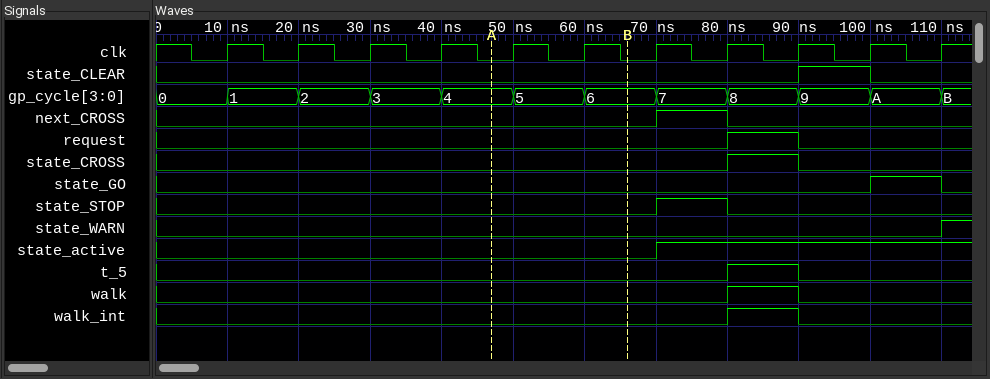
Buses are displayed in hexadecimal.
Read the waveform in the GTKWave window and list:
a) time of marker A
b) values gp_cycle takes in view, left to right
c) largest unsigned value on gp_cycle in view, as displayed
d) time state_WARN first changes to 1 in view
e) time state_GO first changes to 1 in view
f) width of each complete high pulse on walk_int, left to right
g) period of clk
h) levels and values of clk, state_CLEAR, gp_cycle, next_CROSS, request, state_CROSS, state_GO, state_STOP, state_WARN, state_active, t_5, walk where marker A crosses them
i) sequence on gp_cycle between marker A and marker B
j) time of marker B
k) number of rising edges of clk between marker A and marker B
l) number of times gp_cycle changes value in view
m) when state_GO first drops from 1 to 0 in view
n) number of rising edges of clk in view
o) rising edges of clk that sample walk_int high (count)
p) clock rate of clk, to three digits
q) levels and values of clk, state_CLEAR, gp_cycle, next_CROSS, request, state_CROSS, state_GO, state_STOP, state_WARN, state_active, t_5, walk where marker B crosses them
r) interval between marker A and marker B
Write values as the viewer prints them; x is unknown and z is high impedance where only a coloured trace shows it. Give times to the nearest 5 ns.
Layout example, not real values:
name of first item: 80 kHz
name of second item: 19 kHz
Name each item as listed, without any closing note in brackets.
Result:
time of marker A: 45 ns
values gp_cycle takes in view, left to right: 0, 1, 2, 3, 4, 5, 6, 7, 8, 9, A, B
largest unsigned value on gp_cycle in view, as displayed: B
time state_WARN first changes to 1 in view: 110 ns
time state_GO first changes to 1 in view: 100 ns
width of each complete high pulse on walk_int, left to right: 10 ns
period of clk: 10 ns
levels and values of clk, state_CLEAR, gp_cycle, next_CROSS, request, state_CROSS, state_GO, state_STOP, state_WARN, state_active, t_5, walk where marker A crosses them: clk=0, state_CLEAR=0, gp_cycle=4, next_CROSS=0, request=0, state_CROSS=0, state_GO=0, state_STOP=0, state_WARN=0, state_active=0, t_5=0, walk=0
sequence on gp_cycle between marker A and marker B: 4, 5, 6
time of marker B: 65 ns
number of rising edges of clk between marker A and marker B: 2
number of times gp_cycle changes value in view: 11
when state_GO first drops from 1 to 0 in view: 110 ns
number of rising edges of clk in view: 11
rising edges of clk that sample walk_int high: 1
clock rate of clk, to three digits: 100 MHz
levels and values of clk, state_CLEAR, gp_cycle, next_CROSS, request, state_CROSS, state_GO, state_STOP, state_WARN, state_active, t_5, walk where marker B crosses them: clk=0, state_CLEAR=0, gp_cycle=6, next_CROSS=0, request=0, state_CROSS=0, state_GO=0, state_STOP=0, state_WARN=0, state_active=0, t_5=0, walk=0
interval between marker A and marker B: 20 ns
